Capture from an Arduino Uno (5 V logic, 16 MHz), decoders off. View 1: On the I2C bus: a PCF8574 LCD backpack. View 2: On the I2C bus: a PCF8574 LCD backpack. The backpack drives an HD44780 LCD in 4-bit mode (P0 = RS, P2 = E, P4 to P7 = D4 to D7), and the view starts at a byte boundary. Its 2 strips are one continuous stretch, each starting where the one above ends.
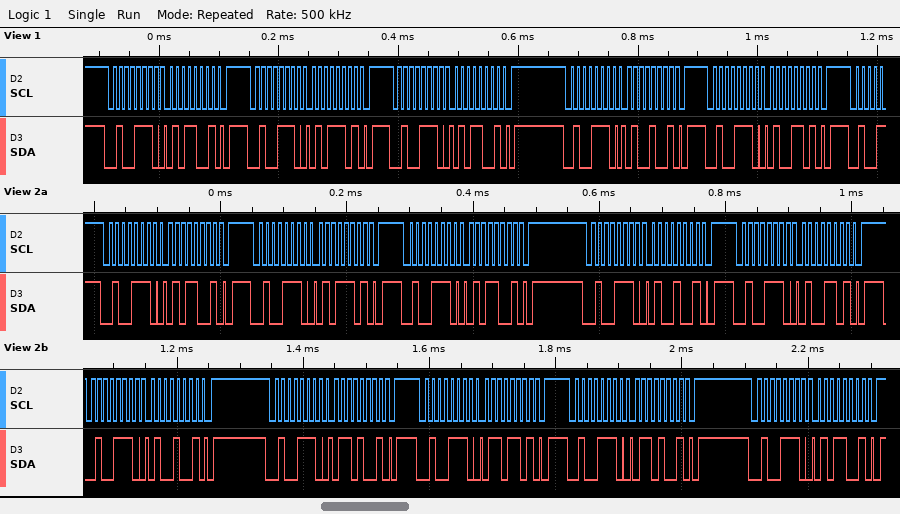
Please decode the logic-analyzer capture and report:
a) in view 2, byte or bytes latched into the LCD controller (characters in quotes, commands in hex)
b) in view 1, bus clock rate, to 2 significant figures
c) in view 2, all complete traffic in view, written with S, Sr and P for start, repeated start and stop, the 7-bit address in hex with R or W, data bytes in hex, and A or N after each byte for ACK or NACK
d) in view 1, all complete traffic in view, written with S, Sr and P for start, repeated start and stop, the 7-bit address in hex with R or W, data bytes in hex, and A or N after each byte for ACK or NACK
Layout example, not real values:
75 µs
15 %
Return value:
'T'
100 kHz
S 27W A 59 A P S 27W A 5D A P S 27W A 59 A P S 27W A 49 A P S 27W A 4D A P S 27W A 49 A P S 27W A 69 A P S 27W A 6D A P S 27W A 69 A P S 27W A 59 A P
S 27W A 59 A P S 27W A 5D A P S 27W A 59 A P S 27W A 49 A P S 27W A 4D A P
